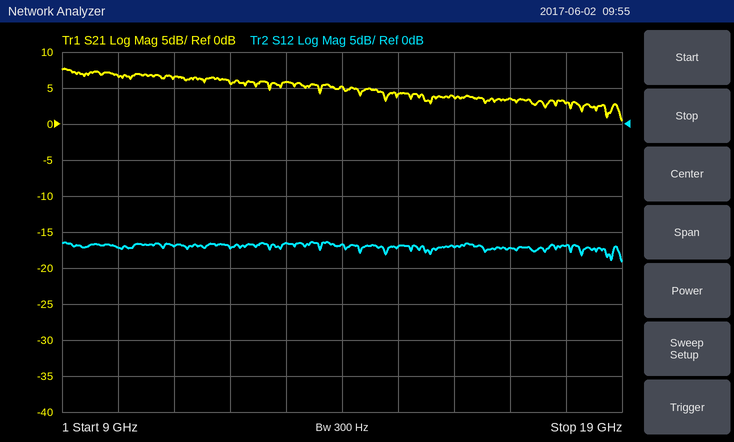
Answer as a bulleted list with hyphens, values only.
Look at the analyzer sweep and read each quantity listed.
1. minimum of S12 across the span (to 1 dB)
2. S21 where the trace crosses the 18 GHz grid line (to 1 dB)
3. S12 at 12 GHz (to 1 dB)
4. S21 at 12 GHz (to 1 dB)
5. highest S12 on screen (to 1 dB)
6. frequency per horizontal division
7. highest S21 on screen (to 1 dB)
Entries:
- -19 dB
- 3 dB
- -17 dB
- 6 dB
- -16 dB
- 1 GHz
- 8 dB
